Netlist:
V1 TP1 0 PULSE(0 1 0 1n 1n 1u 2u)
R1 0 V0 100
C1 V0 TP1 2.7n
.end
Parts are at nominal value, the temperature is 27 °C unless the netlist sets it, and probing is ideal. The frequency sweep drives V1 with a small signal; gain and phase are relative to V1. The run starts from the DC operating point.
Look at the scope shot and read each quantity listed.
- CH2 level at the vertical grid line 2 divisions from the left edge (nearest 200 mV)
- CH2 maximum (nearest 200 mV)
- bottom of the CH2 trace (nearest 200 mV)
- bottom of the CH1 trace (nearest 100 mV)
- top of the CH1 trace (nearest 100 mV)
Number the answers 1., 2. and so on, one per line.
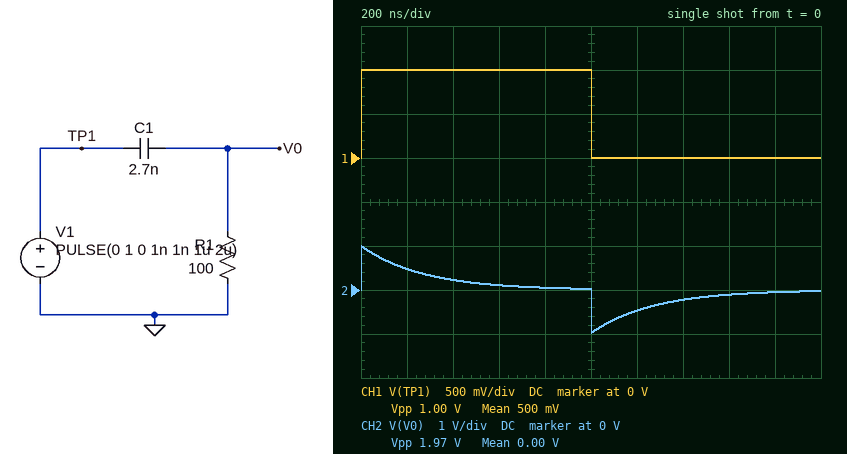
1. 200 mV
2. 1.0 V
3. -1.0 V
4. 0 V
5. 1.0 V
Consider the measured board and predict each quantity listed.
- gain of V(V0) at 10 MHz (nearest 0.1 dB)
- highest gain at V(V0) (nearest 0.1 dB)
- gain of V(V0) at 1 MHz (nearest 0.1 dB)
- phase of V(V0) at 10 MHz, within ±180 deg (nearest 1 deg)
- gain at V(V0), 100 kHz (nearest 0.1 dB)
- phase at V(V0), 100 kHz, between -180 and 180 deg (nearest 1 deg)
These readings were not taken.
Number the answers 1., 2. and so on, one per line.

1. 0 dB
2. 0 dB
3. -1.3 dB
4. 3 deg
5. -15.5 dB
6. 80 deg
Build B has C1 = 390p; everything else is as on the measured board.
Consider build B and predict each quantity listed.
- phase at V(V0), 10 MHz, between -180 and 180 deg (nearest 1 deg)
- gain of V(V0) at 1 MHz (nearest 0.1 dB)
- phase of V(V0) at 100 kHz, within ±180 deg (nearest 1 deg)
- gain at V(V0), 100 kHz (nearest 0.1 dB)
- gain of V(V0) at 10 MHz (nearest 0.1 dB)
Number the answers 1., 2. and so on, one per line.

1. 22 deg
2. -12.5 dB
3. 89 deg
4. -32.2 dB
5. -0.7 dB
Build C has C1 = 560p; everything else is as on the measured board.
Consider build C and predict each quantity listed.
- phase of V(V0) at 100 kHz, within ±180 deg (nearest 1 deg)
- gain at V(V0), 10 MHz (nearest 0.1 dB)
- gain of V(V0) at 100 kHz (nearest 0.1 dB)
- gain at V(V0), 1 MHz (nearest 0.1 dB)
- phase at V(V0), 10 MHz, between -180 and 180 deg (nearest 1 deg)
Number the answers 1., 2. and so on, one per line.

1. 88 deg
2. -0.3 dB
3. -29.1 dB
4. -9.6 dB
5. 16 deg
